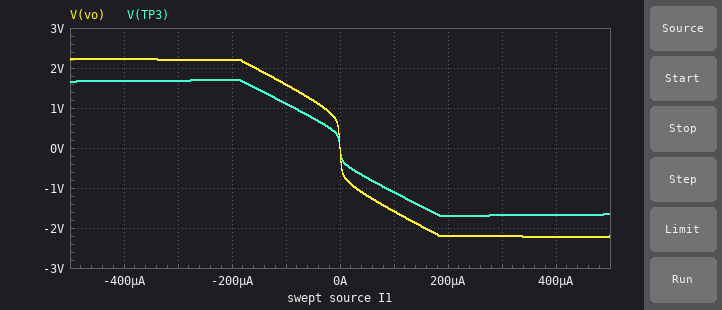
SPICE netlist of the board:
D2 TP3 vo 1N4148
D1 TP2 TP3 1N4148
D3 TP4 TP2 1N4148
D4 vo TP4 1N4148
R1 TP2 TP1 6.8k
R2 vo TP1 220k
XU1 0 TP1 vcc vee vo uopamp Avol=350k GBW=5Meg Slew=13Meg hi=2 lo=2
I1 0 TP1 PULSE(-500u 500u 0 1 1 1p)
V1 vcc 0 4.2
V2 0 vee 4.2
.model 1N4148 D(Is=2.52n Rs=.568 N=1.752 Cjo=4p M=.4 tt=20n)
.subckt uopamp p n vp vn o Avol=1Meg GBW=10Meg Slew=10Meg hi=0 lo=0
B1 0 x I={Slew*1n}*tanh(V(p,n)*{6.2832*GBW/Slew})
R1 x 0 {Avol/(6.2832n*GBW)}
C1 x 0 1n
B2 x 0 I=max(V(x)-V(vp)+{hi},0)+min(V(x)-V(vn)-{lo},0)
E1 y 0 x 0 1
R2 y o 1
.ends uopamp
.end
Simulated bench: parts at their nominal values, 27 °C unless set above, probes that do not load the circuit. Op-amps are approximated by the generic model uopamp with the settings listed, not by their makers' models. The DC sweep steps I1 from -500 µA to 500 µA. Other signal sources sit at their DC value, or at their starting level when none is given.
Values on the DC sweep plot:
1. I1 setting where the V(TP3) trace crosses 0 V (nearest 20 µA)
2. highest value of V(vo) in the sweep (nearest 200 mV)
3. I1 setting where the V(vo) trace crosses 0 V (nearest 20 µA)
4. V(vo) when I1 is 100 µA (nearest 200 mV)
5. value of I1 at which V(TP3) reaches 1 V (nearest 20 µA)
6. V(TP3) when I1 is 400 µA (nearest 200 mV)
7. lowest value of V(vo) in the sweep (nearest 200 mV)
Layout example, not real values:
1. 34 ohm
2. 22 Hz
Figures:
1. 0 A
2. 2.2 V
3. 0 A
4. -1.6 V
5. -80 µA
6. -1.6 V
7. -2.2 V
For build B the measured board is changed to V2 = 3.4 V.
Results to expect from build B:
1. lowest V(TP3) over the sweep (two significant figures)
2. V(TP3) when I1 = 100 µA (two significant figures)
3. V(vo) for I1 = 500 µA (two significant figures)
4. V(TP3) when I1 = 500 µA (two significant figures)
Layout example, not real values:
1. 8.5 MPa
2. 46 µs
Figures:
1. -940 mV
2. -930 mV
3. -1.4 V
4. -860 mV
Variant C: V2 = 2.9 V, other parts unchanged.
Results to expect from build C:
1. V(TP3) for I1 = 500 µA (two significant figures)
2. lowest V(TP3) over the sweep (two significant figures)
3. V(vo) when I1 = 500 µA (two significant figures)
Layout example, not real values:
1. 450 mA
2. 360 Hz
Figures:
1. -360 mV
2. -500 mV
3. -910 mV
